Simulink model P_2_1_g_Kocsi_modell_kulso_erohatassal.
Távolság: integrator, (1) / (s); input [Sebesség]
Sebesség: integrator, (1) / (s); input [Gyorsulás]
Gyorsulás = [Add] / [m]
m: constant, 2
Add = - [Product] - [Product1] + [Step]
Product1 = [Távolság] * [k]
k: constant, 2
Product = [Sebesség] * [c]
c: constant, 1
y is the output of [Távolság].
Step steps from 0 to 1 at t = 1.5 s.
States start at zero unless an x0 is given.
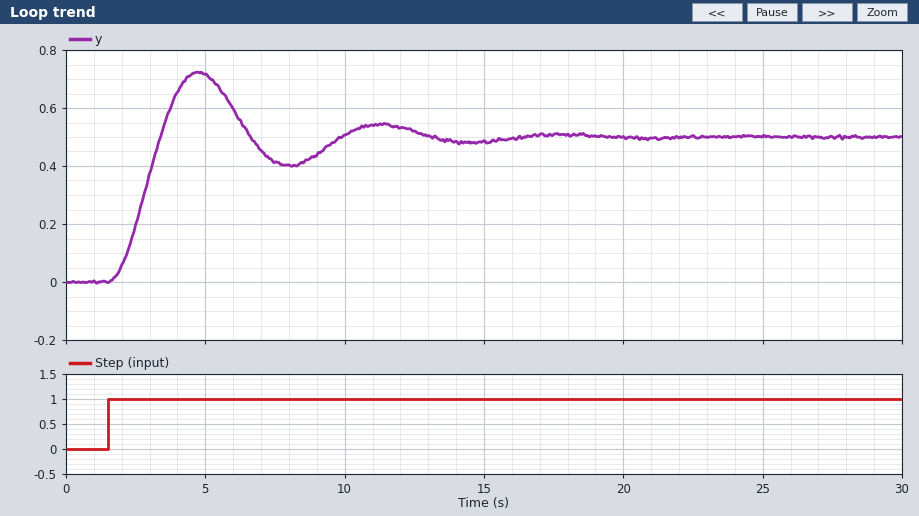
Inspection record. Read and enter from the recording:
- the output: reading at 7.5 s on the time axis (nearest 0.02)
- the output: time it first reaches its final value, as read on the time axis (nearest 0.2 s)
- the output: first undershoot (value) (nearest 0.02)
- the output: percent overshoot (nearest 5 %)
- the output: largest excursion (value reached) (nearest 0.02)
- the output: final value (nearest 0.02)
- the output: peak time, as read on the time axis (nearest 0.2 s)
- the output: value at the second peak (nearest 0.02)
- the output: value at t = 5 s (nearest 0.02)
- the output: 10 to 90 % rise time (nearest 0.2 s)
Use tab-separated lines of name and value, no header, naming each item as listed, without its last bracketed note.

the output: reading at 7.5 s on the time axis	0.42
the output: time it first reaches its final value, as read on the time axis	3.4 s
the output: first undershoot (value)	0.40
the output: percent overshoot	45 %
the output: largest excursion (value reached)	0.72
the output: final value	0.50
the output: peak time, as read on the time axis	4.8 s
the output: value at the second peak	0.54
the output: value at t = 5 s	0.72
the output: 10 to 90 % rise time	1.2 s
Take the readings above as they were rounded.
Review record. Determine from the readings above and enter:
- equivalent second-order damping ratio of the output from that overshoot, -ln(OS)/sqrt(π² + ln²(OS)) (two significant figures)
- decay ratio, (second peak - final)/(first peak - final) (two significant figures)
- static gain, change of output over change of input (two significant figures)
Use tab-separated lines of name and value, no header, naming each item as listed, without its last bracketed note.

equivalent second-order damping ratio of the output from that overshoot, -ln(OS)/sqrt(π² + ln²(OS))	0.25
decay ratio, (second peak - final)/(first peak - final)	0.18
static gain, change of output over change of input	0.50
